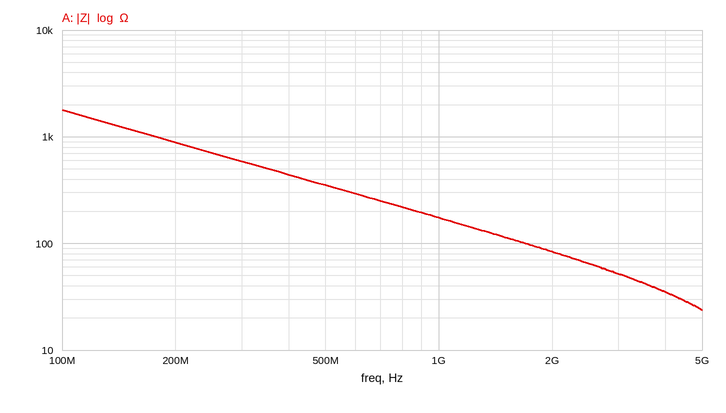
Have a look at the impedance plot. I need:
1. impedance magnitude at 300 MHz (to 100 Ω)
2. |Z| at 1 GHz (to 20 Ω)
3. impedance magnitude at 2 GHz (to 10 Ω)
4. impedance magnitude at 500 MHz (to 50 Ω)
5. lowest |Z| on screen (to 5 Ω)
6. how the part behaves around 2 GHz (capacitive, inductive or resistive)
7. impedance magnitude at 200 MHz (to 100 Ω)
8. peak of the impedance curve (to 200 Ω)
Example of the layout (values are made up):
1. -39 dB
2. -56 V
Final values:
1. 600 Ω
2. 180 Ω
3. 80 Ω
4. 350 Ω
5. 25 Ω
6. capacitive
7. 900 Ω
8. 1.8 kΩ
